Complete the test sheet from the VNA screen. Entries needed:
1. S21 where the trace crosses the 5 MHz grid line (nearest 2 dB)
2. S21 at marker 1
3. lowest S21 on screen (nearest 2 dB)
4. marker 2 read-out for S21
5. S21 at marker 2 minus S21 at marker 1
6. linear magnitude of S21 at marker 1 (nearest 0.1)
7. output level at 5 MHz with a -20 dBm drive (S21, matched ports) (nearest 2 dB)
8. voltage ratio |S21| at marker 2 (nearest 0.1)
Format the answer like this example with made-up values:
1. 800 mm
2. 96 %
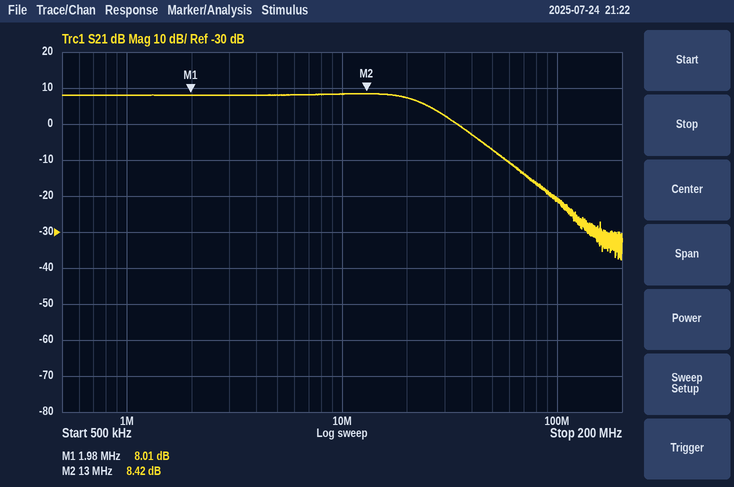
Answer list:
1. 8 dB
2. 8.01 dB
3. -38 dB
4. 8.42 dB
5. 0.41 dB
6. 2.5
7. -12 dBm
8. 2.6
